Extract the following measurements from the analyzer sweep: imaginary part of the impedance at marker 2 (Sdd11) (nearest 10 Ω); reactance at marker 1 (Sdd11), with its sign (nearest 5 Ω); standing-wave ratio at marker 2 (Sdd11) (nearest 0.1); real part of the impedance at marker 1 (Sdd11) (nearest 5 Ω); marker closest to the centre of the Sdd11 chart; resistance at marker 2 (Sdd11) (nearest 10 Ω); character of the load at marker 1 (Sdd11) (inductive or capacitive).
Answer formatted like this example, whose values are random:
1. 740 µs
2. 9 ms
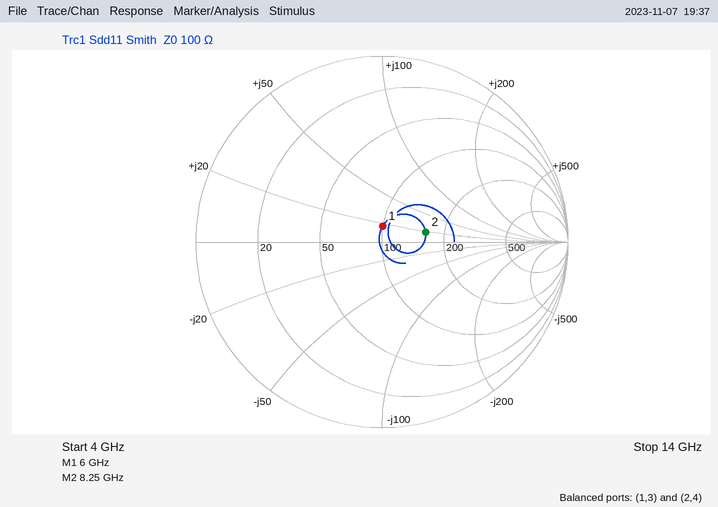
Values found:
1. +20 Ω
2. +15 Ω
3. 1.6
4. 100 Ω
5. marker 1
6. 160 Ω
7. inductive
